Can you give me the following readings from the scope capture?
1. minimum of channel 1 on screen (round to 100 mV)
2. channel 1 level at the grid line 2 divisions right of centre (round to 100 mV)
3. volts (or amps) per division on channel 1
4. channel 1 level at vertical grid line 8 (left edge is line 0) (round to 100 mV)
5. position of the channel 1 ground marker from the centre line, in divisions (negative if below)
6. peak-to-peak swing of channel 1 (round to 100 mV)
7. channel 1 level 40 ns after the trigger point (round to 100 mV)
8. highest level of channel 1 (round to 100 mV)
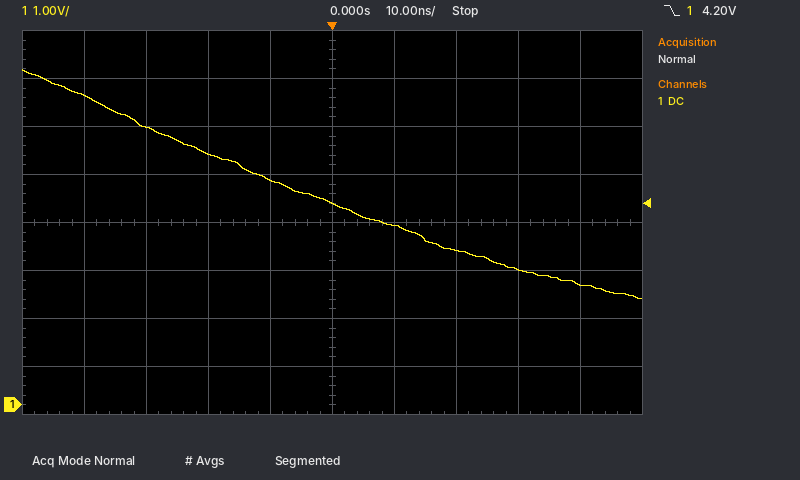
2.2 V
3.2 V
1 V
2.8 V
-3.8 div
4.8 V
2.5 V
7.0 V
